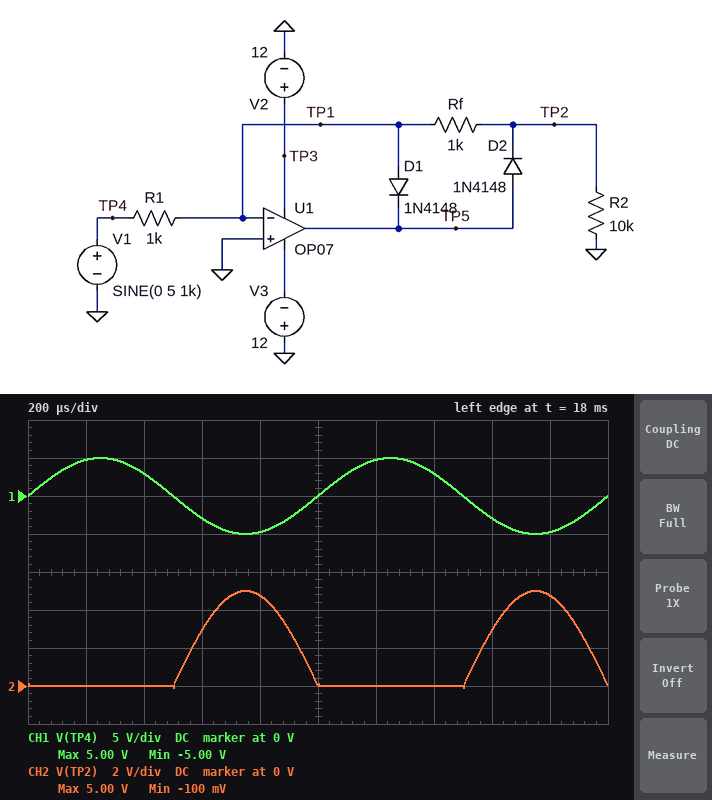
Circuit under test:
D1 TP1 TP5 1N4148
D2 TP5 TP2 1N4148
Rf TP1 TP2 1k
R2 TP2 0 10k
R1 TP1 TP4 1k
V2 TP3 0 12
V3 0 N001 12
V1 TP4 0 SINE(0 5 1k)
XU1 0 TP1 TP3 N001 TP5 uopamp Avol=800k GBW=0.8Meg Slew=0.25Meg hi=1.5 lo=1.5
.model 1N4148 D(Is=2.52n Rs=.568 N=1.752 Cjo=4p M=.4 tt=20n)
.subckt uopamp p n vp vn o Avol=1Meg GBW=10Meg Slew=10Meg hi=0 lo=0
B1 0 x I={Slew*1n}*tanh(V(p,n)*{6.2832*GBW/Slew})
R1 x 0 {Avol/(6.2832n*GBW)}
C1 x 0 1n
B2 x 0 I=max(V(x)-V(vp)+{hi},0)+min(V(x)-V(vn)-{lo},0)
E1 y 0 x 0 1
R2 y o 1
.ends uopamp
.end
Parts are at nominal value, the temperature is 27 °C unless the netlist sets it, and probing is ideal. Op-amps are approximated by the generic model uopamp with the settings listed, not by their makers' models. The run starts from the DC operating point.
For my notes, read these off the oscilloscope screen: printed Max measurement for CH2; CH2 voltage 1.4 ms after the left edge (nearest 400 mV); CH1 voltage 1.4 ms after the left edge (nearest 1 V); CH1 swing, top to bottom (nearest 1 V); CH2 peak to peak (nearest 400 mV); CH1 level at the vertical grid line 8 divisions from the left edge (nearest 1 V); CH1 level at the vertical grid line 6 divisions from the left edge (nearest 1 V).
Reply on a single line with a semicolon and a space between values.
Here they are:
5.00 V; 0 V; 3 V; 10 V; 5.2 V; -3 V; 5 V
